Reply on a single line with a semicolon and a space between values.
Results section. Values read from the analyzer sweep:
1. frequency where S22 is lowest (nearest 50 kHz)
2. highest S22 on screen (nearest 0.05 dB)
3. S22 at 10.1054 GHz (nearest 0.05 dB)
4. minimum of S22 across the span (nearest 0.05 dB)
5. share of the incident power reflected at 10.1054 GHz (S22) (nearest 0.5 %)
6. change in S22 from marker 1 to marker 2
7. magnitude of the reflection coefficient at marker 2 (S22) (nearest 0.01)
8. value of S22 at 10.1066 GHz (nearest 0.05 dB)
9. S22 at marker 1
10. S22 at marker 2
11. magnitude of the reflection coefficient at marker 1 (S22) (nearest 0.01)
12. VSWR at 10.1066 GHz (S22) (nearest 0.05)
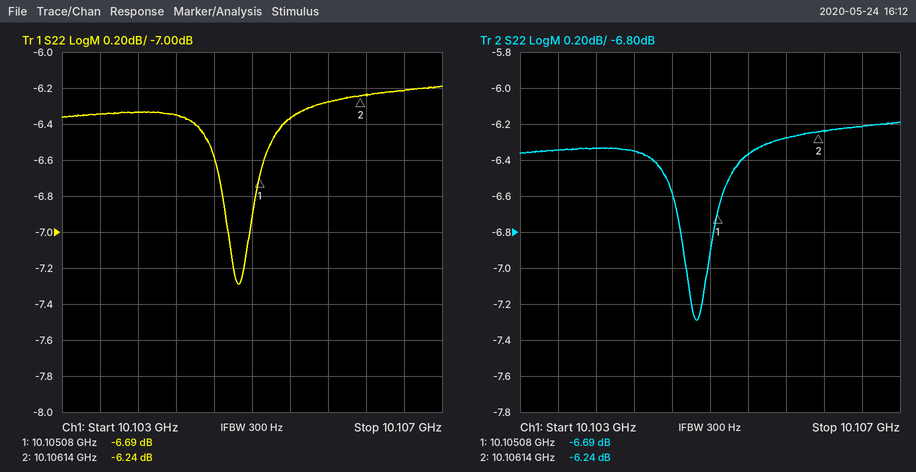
10.10485 GHz; -6.20 dB; -6.35 dB; -7.30 dB; 23.0 %; 0.45 dB; 0.49; -6.20 dB; -6.69 dB; -6.24 dB; 0.46; 2.90
